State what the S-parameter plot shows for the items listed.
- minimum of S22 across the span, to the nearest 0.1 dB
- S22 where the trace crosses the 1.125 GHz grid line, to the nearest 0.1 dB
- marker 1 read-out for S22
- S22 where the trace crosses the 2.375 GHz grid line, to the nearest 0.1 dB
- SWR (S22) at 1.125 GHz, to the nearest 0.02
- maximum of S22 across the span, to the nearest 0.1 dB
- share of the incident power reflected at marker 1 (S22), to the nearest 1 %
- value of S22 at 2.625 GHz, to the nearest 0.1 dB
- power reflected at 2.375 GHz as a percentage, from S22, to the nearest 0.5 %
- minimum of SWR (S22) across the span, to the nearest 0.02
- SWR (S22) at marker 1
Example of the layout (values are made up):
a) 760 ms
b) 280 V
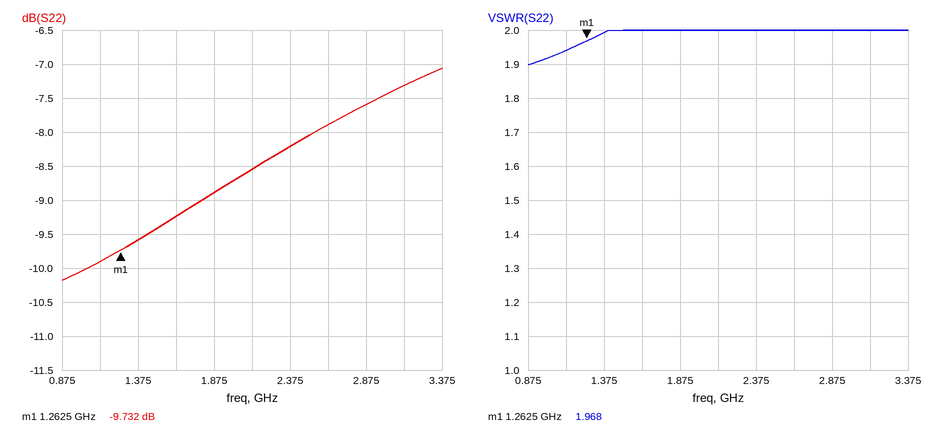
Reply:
a) -10.2 dB
b) -9.9 dB
c) -9.732 dB
d) -8.2 dB
e) 1.94
f) -7.1 dB
g) 11 %
h) -7.9 dB
i) 15.0 %
j) 1.90
k) 1.968
